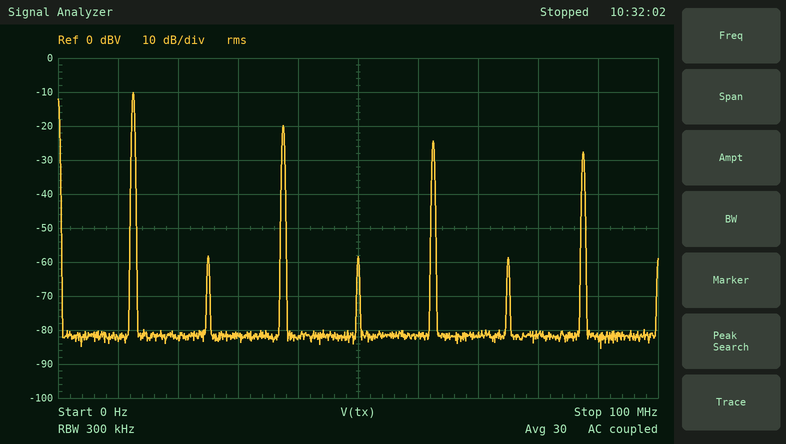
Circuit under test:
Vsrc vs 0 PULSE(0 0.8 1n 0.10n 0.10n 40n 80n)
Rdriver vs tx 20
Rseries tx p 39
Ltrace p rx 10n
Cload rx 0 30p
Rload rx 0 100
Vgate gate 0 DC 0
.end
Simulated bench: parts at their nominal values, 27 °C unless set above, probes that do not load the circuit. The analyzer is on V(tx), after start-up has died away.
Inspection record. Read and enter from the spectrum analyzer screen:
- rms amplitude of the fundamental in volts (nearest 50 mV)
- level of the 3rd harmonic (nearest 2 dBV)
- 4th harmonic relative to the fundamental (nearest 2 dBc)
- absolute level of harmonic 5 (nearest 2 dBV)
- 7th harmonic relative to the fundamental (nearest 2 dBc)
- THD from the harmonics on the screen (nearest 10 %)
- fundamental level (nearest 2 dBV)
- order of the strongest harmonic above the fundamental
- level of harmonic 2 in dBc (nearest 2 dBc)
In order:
300 mV
-20 dBV
-48 dBc
-24 dBV
-18 dBc
40 %
-10 dBV
3
-48 dBc
